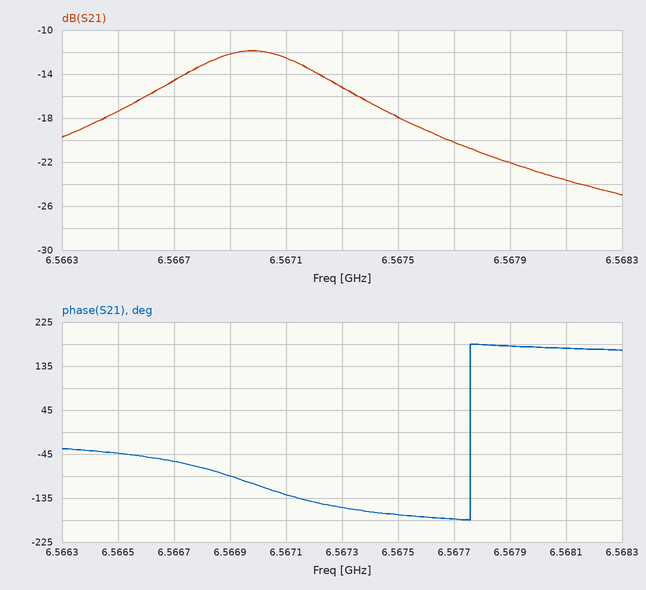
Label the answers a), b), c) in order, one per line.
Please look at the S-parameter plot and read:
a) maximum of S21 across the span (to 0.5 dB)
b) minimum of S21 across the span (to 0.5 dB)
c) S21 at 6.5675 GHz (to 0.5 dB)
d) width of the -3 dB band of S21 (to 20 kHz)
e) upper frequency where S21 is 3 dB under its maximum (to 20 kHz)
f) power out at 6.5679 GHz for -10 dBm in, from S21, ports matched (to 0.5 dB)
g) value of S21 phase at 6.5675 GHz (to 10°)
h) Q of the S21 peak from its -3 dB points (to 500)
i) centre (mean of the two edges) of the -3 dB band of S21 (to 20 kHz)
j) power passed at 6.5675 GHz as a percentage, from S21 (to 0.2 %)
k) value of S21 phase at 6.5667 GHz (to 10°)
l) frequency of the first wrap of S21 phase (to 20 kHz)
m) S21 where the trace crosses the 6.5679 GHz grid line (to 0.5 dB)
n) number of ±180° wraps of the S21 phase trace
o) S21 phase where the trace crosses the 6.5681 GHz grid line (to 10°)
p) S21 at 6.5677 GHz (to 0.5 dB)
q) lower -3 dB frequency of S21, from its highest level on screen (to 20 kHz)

a) -12.0 dB
b) -25.0 dB
c) -18.0 dB
d) 600 kHz
e) 6.56728 GHz
f) -32.0 dBm
g) -170°
h) 11000
i) 6.56698 GHz
j) 1.6 %
k) -60°
l) 6.56776 GHz
m) -22.0 dB
n) 1
o) 170°
p) -20.0 dB
q) 6.56668 GHz
